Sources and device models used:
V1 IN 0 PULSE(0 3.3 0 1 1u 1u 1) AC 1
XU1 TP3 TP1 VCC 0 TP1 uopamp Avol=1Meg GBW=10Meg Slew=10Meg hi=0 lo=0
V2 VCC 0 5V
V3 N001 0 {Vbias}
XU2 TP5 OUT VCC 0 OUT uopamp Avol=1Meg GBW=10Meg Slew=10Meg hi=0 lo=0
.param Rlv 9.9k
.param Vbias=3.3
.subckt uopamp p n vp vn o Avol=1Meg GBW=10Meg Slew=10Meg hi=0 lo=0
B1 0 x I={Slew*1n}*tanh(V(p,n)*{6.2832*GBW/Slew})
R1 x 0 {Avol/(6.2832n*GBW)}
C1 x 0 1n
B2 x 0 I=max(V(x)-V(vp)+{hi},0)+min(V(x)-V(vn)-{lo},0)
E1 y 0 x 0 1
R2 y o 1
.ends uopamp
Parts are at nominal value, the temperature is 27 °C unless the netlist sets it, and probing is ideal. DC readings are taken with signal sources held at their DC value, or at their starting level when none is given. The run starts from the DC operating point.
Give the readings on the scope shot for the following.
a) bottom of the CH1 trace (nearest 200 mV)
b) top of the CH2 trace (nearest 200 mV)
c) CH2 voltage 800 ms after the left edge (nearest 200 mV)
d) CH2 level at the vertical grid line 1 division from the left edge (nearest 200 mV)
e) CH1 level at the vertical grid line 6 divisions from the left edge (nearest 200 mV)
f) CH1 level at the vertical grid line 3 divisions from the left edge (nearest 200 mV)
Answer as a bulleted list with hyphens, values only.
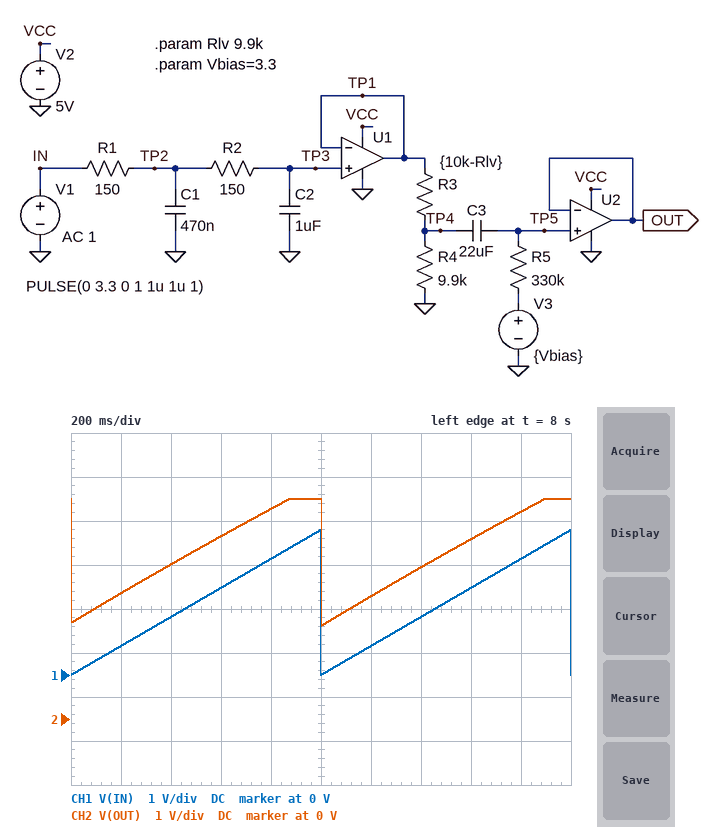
- 0 V
- 5.0 V
- 4.8 V
- 2.8 V
- 600 mV
- 2.0 V
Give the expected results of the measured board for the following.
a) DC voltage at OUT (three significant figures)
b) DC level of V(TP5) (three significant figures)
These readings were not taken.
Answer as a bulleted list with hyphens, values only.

- 3.30 V
- 3.30 V
